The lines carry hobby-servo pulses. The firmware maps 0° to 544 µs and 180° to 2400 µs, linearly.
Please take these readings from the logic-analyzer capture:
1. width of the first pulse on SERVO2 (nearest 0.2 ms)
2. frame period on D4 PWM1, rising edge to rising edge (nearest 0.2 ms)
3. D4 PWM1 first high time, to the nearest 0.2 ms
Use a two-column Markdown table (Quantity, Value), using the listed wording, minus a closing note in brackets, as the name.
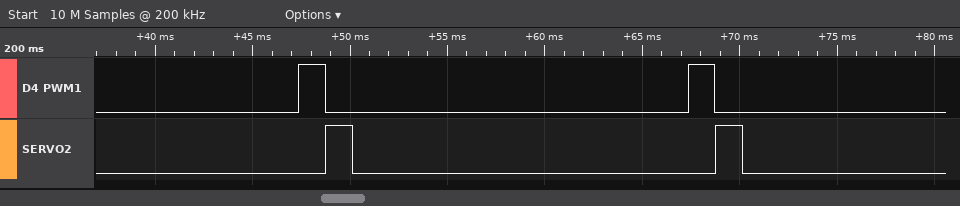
| Quantity | Value |
|---|---|
| width of the first pulse on SERVO2 | 1.4 ms |
| frame period on D4 PWM1, rising edge to rising edge | 20.0 ms |
| D4 PWM1 first high time, to the nearest 0.2 ms | 1.4 ms |
